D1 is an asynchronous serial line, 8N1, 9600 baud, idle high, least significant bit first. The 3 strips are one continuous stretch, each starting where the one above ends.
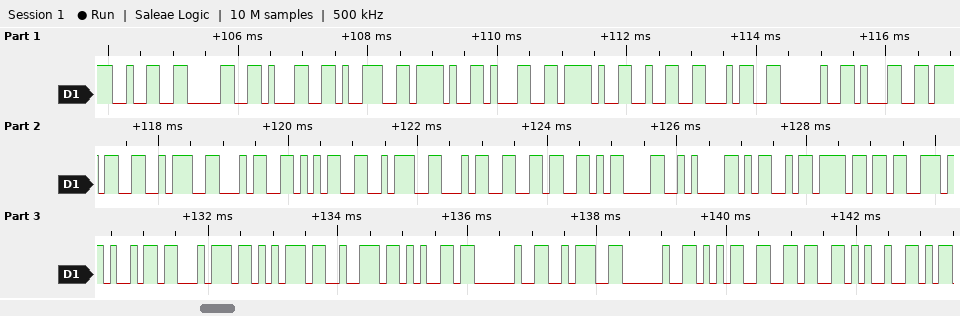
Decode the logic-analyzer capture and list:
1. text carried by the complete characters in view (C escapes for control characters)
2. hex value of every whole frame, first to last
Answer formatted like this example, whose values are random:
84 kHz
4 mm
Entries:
"2019/1/24 17:45:46\r\nMositure : 56%"
32 30 31 39 2F 31 2F 32 34 20 31 37 3A 34 35 3A 34 36 0D 0A 4D 6F 73 69 74 75 72 65 20 3A 20 35 36 25
